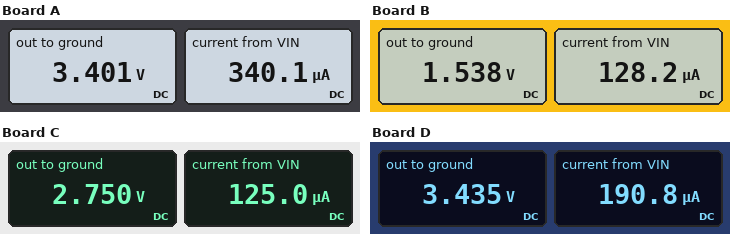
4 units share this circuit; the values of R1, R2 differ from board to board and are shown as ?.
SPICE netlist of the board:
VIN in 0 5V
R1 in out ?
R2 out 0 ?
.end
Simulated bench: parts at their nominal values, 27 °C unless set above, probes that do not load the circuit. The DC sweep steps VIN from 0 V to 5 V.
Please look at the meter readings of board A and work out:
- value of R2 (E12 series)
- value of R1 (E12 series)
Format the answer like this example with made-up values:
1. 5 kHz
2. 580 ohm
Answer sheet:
1. 10 kΩ
2. 4.7 kΩ
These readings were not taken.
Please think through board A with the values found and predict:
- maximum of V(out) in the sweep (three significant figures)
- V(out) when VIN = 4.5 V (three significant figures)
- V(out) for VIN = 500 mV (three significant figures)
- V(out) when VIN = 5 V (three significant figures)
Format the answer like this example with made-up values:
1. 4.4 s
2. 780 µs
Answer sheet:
1. 3.40 V
2. 3.06 V
3. 340 mV
4. 3.40 V
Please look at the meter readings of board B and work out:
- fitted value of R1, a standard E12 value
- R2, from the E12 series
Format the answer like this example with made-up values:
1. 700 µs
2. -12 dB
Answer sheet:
1. 27 kΩ
2. 12 kΩ
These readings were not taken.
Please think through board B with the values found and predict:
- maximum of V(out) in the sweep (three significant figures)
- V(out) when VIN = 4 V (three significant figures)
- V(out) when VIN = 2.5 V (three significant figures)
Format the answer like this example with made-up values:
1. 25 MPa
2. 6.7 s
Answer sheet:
1. 1.54 V
2. 1.23 V
3. 769 mV
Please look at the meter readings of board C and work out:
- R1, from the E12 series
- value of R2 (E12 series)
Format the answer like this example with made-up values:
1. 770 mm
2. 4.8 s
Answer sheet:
1. 18 kΩ
2. 22 kΩ
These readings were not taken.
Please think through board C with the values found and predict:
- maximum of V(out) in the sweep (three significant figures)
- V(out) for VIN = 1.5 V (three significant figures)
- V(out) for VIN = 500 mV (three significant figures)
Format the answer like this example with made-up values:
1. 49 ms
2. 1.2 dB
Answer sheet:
1. 2.75 V
2. 825 mV
3. 275 mV
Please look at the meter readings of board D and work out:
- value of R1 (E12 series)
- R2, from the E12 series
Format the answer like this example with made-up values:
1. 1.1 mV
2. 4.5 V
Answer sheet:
1. 8.2 kΩ
2. 18 kΩ
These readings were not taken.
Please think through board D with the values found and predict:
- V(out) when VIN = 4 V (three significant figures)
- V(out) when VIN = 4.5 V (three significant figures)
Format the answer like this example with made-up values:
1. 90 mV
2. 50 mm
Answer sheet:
1. 2.75 V
2. 3.09 V
